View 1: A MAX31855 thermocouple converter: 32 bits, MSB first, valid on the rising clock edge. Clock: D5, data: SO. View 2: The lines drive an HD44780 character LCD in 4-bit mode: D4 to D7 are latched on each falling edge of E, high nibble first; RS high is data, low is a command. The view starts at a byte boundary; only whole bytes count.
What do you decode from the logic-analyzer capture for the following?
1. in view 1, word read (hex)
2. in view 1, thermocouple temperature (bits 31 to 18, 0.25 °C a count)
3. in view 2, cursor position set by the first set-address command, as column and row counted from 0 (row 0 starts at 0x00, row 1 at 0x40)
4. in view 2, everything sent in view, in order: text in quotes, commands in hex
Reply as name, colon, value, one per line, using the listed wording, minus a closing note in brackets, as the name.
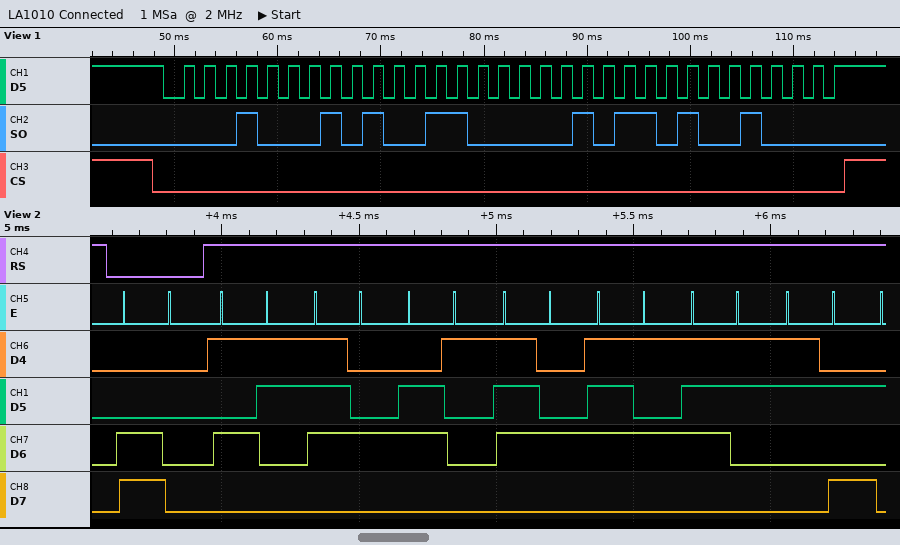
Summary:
in view 1, word read: 0x114C1690
in view 1, thermocouple temperature: 276.75 °C
in view 2, cursor position set by the first set-address command, as column and row counted from 0: column 0, row 1
in view 2, everything sent in view, in order: text in quotes, commands in hex: 0xC0 "Status:"
